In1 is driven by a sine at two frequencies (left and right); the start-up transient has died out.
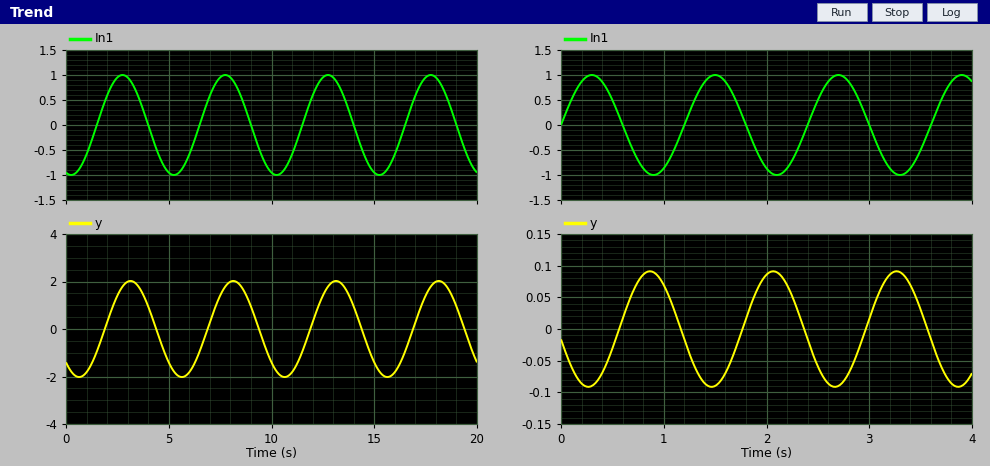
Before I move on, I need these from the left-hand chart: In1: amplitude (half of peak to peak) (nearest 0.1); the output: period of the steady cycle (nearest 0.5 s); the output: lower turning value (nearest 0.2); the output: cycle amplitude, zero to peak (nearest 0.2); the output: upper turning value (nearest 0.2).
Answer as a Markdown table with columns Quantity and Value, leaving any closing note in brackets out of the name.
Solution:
| Quantity | Value |
|---|---|
| In1: amplitude (half of peak to peak) | 1.0 |
| the output: period of the steady cycle | 5.0 s |
| the output: lower turning value | -2.0 |
| the output: cycle amplitude, zero to peak | 2.0 |
| the output: upper turning value | 2.0 |
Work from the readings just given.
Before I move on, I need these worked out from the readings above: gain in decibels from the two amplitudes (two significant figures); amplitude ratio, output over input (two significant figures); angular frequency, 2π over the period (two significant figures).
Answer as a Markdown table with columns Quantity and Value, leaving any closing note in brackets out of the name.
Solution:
| Quantity | Value |
|---|---|
| gain in decibels from the two amplitudes | 6.0 dB |
| amplitude ratio, output over input | 2.0 |
| angular frequency, 2π over the period | 1.3 rad/s |
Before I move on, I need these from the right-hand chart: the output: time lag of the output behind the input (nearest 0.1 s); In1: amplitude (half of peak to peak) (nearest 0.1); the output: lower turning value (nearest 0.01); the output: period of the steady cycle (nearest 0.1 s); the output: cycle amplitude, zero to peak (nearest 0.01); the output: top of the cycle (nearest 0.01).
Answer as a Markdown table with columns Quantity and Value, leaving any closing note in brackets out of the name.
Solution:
| Quantity | Value |
|---|---|
| the output: time lag of the output behind the input | 0.6 s |
| In1: amplitude (half of peak to peak) | 1.0 |
| the output: lower turning value | -0.09 |
| the output: period of the steady cycle | 1.2 s |
| the output: cycle amplitude, zero to peak | 0.09 |
| the output: top of the cycle | 0.09 |
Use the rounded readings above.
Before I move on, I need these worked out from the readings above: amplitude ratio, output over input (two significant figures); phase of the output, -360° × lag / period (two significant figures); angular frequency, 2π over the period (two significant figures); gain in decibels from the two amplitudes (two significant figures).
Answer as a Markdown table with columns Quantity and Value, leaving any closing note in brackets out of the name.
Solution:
| Quantity | Value |
|---|---|
| amplitude ratio, output over input | 0.090 |
| phase of the output, -360° × lag / period | -180° |
| angular frequency, 2π over the period | 5.2 rad/s |
| gain in decibels from the two amplitudes | -21 dB |
